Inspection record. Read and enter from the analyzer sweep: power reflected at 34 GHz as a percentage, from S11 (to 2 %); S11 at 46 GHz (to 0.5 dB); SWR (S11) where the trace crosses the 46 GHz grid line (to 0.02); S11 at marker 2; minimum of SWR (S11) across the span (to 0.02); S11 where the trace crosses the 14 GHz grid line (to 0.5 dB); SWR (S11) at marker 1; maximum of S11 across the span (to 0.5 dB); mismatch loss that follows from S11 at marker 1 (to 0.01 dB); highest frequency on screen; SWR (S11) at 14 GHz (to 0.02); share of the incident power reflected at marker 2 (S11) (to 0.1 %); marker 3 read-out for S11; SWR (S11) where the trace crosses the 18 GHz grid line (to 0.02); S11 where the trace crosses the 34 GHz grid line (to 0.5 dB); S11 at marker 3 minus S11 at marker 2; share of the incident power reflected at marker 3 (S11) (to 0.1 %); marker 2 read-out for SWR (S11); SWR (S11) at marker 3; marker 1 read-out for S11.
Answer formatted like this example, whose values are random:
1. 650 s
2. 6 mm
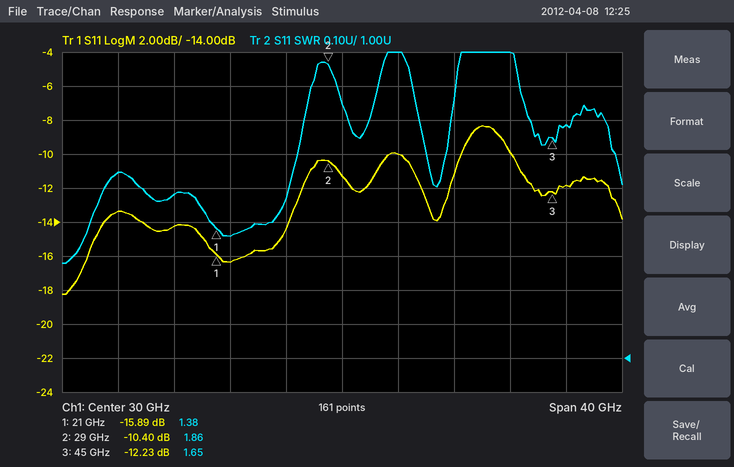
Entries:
1. 10 %
2. -12.0 dB
3. 1.68
4. -10.40 dB
5. 1.28
6. -13.5 dB
7. 1.38
8. -8.5 dB
9. 0.11 dB
10. 50 GHz
11. 1.54
12. 9.1 %
13. -12.23 dB
14. 1.48
15. -10.0 dB
16. -1.83 dB
17. 6.0 %
18. 1.86
19. 1.65
20. -15.89 dB
